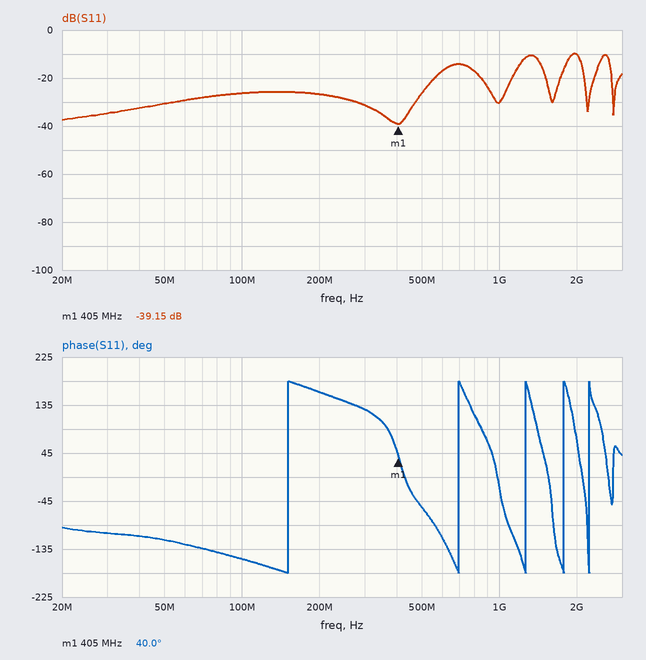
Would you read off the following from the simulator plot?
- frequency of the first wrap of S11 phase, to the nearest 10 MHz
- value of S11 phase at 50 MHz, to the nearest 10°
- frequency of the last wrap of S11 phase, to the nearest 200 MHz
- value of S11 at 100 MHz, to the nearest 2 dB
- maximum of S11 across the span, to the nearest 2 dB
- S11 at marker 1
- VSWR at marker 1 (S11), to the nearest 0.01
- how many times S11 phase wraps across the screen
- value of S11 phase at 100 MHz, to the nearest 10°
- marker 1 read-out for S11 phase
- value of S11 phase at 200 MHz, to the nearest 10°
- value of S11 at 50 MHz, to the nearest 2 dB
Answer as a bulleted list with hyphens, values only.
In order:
- 150 MHz
- -120°
- 2.2 GHz
- -26 dB
- -10 dB
- -39.15 dB
- 1.02
- 5
- -150°
- 40.0°
- 160°
- -30 dB
